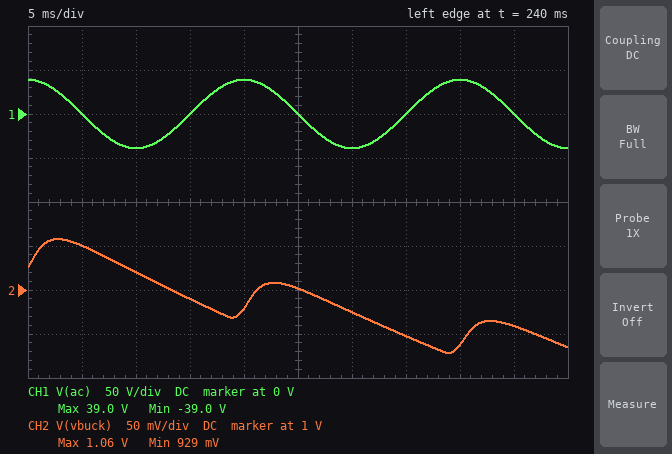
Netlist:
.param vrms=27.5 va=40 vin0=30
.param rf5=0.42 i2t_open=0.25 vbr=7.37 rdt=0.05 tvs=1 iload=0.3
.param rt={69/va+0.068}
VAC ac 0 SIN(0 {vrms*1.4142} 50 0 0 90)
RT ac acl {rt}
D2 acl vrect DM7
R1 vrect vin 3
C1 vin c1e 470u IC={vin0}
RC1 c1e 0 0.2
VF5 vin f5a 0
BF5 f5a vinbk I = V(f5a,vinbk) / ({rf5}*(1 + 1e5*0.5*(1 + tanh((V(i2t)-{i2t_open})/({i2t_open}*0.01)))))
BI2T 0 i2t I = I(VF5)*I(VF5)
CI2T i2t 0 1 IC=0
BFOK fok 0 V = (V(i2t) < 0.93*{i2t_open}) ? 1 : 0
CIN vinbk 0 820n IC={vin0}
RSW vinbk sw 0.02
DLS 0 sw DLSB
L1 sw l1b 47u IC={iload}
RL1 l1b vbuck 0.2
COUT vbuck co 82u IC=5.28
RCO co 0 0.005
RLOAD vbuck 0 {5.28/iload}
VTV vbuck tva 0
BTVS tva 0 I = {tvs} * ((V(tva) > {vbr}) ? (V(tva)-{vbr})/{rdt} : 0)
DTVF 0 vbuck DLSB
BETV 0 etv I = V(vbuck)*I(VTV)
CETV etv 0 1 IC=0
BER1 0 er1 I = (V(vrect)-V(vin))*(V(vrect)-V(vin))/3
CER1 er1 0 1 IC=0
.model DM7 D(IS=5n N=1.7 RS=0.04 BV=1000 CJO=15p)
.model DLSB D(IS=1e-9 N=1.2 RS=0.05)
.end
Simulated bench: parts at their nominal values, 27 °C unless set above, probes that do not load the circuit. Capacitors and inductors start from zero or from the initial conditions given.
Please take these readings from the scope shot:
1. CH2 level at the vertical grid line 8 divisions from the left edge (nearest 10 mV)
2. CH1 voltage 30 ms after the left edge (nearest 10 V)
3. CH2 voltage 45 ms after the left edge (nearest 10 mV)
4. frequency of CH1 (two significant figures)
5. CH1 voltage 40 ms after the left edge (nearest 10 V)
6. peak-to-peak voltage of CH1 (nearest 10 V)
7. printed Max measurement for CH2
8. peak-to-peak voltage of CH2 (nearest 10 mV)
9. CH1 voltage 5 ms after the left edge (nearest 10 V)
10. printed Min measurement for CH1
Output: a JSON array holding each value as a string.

["940 mV", "-40 V", "960 mV", "50 Hz", "40 V", "80 V", "1.06 V", "130 mV", "0 V", "-39.0 V"]
